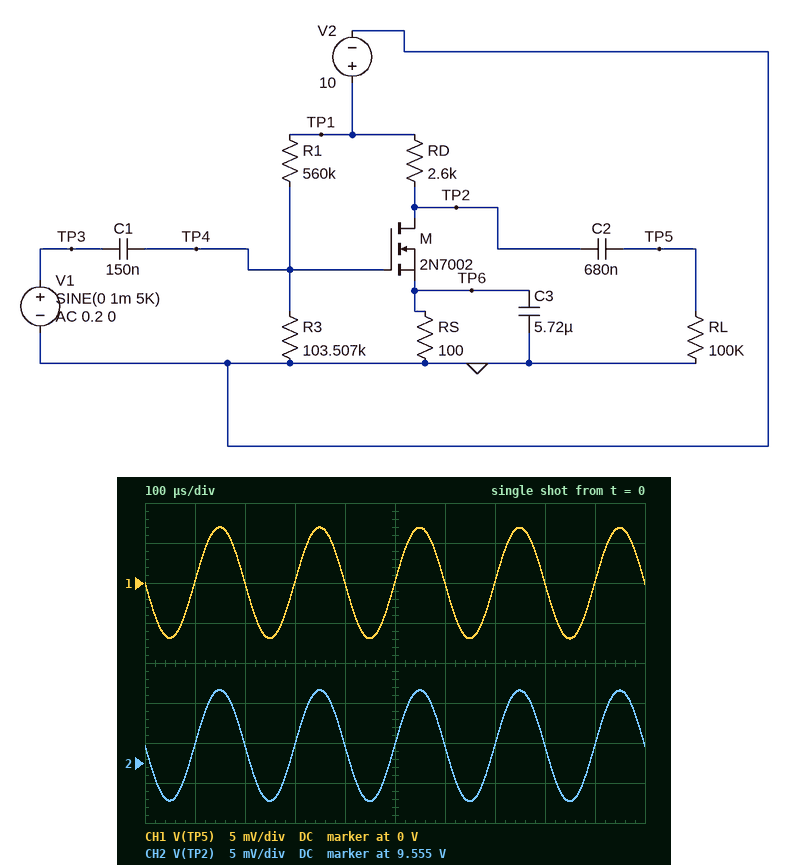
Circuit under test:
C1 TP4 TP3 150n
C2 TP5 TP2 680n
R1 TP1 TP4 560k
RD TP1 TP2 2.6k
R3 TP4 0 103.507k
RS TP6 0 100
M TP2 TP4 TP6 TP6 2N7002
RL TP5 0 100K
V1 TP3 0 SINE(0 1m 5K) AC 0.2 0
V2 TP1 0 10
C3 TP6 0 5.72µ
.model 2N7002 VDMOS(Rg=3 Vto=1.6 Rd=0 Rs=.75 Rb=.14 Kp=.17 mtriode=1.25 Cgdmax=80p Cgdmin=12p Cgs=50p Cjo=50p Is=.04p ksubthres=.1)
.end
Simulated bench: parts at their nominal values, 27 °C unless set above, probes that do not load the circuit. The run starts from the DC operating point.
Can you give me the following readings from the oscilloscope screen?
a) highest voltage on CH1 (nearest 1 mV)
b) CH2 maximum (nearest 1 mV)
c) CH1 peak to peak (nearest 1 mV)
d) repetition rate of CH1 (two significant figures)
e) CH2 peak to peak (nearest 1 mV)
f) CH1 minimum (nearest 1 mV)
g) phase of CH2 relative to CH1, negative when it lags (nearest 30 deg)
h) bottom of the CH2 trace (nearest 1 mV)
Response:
7 mV
9.564 V
14 mV
5.0 kHz
14 mV
-7 mV
0 deg
9.550 V
